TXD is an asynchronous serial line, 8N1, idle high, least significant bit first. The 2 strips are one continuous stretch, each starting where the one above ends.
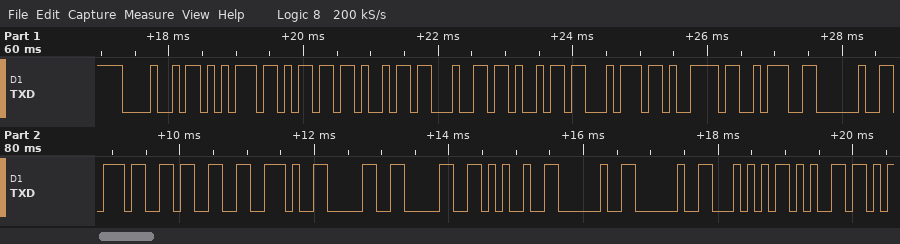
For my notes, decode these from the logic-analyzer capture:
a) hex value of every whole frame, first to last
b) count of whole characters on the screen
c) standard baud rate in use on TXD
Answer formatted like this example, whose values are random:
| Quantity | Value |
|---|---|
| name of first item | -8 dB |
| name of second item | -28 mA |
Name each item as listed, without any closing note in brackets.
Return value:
| Quantity | Value |
|---|---|
| hex value of every whole frame, first to last | 0x48 0x75 0x6D 0x69 0x64 0x69 0x74 0x79 0x3A 0x20 0x37 0x33 0x2E 0x30 0x30 0x25 0x20 0x20 0x54 0x65 |
| count of whole characters on the screen | 20 |
| standard baud rate in use on TXD | 9600 baud |
